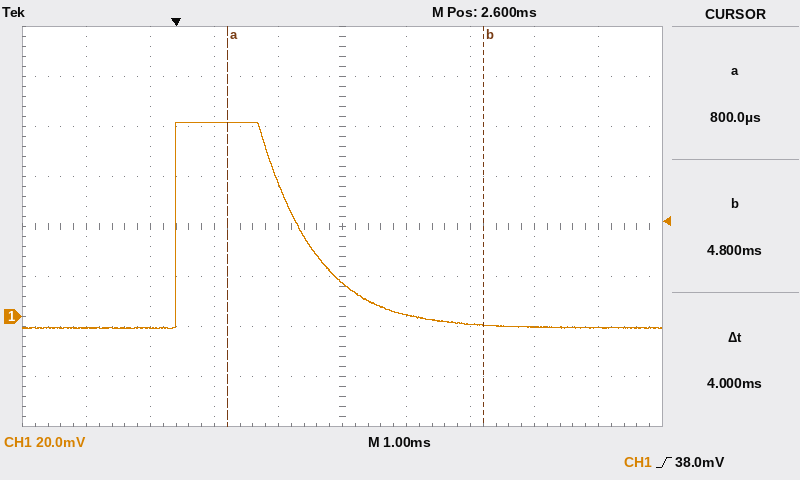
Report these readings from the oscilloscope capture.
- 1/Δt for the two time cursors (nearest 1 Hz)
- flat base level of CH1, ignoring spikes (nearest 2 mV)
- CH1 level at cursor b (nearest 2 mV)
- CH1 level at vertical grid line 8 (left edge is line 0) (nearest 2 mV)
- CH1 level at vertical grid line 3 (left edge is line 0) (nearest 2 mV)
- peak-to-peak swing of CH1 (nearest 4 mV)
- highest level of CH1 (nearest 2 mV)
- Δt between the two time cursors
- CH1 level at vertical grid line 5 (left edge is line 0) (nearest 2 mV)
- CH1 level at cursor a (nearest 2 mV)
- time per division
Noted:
250 Hz
-4 mV
-4 mV
-4 mV
78 mV
84 mV
78 mV
4 ms
14 mV
78 mV
1 ms
